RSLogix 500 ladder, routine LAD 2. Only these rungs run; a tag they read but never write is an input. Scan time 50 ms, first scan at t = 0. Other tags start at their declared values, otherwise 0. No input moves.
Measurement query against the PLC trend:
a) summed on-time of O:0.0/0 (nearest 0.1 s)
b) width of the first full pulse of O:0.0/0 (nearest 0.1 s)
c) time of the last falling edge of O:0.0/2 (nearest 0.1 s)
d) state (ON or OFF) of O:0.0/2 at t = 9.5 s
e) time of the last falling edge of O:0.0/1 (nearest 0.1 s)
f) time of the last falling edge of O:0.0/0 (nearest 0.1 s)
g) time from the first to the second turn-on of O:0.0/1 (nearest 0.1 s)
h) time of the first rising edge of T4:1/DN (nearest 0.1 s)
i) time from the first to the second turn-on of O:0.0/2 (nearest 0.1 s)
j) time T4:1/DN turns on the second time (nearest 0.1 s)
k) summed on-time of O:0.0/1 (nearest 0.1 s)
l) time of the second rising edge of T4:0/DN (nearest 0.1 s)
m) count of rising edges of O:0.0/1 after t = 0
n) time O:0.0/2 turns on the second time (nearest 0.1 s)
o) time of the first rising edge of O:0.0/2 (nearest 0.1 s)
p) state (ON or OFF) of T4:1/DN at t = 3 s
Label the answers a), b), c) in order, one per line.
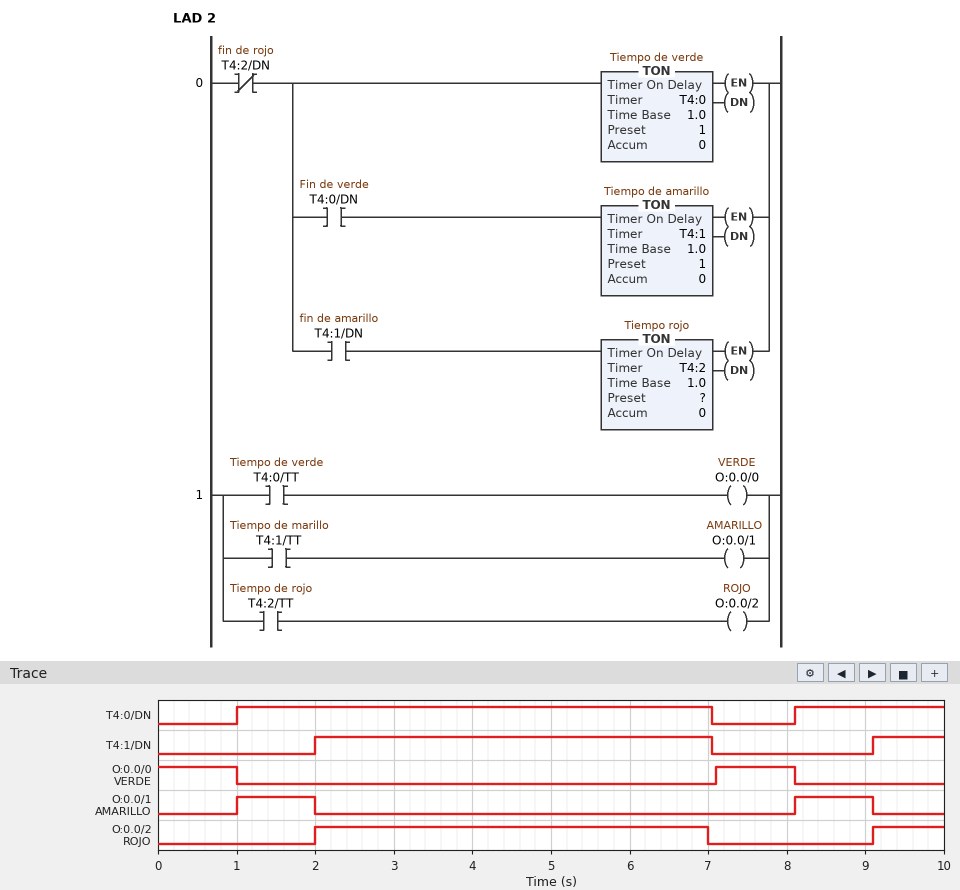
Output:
a) 2.0 s
b) 1.0 s
c) 7.0 s
d) ON
e) 9.1 s
f) 8.1 s
g) 7.1 s
h) 2.0 s
i) 7.1 s
j) 9.1 s
k) 2.0 s
l) 8.1 s
m) 2
n) 9.1 s
o) 2.0 s
p) ON
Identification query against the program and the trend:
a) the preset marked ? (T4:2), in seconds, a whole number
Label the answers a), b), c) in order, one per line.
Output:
a) 5 s
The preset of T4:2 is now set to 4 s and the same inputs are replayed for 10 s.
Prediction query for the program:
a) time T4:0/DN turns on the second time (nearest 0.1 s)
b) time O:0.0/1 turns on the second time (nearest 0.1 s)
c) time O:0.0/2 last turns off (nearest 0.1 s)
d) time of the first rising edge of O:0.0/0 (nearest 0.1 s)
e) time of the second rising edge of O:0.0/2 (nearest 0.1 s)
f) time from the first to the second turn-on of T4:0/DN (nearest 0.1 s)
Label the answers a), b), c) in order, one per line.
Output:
a) 7.1 s
b) 7.1 s
c) 6.0 s
d) 6.1 s
e) 8.1 s
f) 6.1 s
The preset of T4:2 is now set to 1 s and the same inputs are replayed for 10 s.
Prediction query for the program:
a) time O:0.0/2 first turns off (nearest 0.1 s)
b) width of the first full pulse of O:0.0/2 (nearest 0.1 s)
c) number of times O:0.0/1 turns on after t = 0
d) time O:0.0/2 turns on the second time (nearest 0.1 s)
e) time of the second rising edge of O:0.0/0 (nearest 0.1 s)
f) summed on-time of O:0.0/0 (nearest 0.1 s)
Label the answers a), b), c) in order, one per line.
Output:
a) 3.0 s
b) 1.0 s
c) 3
d) 5.1 s
e) 6.2 s
f) 3.7 s
